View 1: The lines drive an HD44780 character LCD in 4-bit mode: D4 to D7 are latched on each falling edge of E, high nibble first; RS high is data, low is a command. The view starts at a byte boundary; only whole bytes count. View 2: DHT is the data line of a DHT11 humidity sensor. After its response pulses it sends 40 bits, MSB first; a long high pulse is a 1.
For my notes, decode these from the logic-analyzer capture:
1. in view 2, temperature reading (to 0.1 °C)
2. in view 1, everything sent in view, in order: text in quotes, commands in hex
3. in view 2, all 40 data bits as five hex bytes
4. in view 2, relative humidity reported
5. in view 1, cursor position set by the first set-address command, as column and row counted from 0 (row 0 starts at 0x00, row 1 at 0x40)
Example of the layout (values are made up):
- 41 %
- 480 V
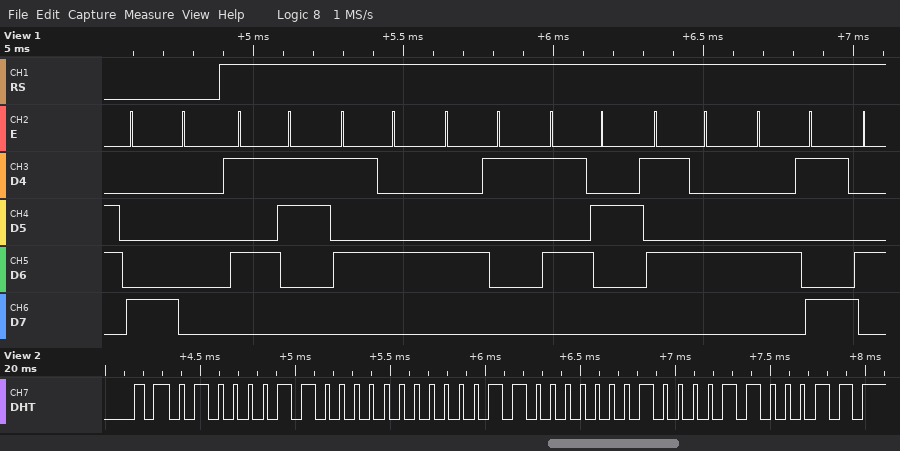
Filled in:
- 24.8 °C
- 0x80 "STARTI"
- 43 00 18 08 63
- 67 %
- column 0, row 0
